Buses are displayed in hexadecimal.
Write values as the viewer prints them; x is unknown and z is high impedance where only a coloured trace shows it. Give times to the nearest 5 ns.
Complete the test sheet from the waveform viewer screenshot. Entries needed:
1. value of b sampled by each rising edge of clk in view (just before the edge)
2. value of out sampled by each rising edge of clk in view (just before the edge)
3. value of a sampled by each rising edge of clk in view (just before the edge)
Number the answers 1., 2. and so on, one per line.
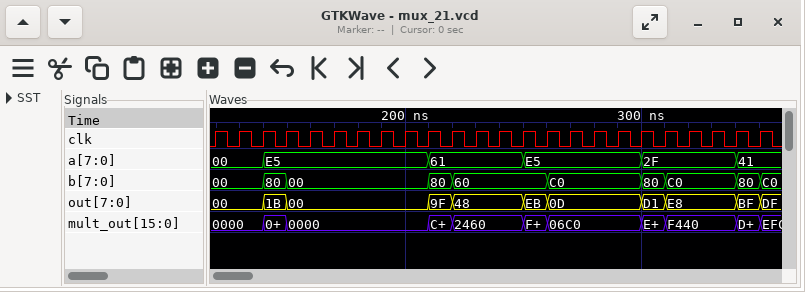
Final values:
1. 00, 00, 00, 80, 00, 00, 00, 00, 00, 00, 80, 60, 60, 60, 60, C0, C0, C0, C0, 80, C0, C0, C0, 80
2. 00, 00, 00, 1B, 00, 00, 00, 00, 00, 00, 9F, 48, 48, 48, EB, 0D, 0D, 0D, 0D, D1, E8, E8, E8, BF
3. 00, 00, 00, E5, E5, E5, E5, E5, E5, E5, 61, 61, 61, 61, E5, E5, E5, E5, E5, 2F, 2F, 2F, 2F, 41
